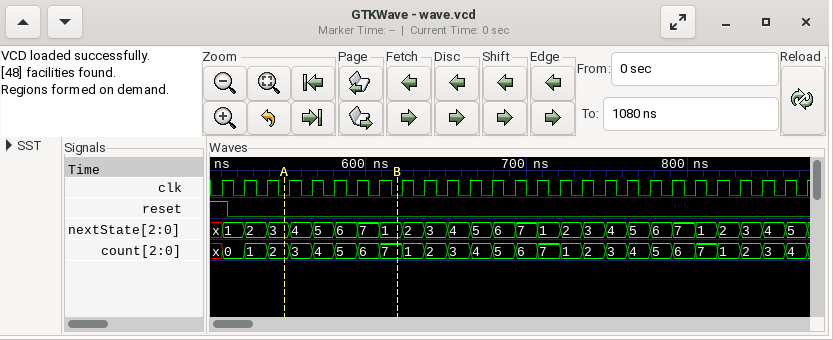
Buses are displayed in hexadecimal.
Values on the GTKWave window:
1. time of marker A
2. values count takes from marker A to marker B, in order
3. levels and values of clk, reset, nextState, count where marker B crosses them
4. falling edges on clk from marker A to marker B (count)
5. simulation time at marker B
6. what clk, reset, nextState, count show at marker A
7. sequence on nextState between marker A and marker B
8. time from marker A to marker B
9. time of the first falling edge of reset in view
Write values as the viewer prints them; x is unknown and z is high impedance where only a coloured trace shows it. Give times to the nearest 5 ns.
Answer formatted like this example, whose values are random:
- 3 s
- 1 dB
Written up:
- 550 ns
- 2, 3, 4, 5, 6, 7
- clk=0, reset=0, nextState=1, count=7
- 5
- 620 ns
- clk=0, reset=0, nextState=3, count=2
- 3, 4, 5, 6, 7, 1
- 70 ns
- 515 ns
